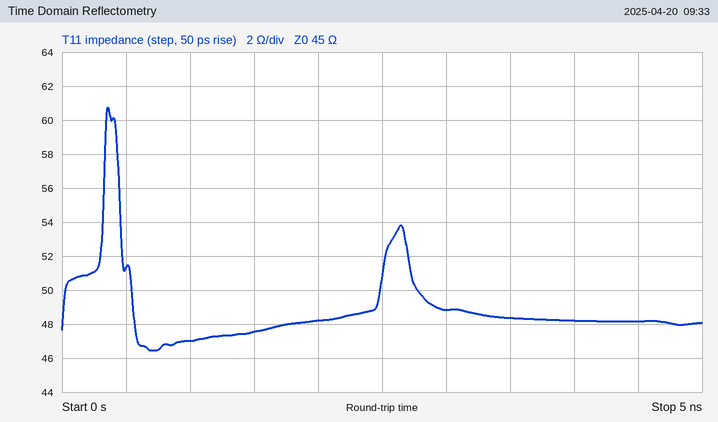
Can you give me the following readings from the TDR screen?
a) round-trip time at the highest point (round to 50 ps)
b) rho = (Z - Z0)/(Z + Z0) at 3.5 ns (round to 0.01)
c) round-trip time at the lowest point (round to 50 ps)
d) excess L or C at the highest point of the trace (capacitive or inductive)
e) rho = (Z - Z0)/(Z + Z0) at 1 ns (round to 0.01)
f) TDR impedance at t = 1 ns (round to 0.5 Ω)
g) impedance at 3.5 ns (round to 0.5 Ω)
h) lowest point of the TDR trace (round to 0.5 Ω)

350 ps
+0.04
700 ps
inductive
+0.02
47.0 Ω
48.5 Ω
46.5 Ω
